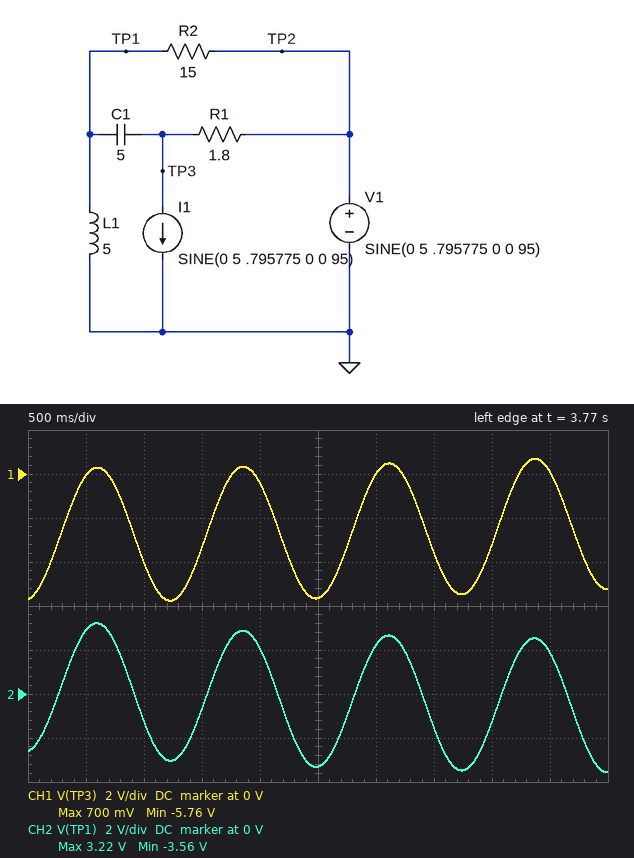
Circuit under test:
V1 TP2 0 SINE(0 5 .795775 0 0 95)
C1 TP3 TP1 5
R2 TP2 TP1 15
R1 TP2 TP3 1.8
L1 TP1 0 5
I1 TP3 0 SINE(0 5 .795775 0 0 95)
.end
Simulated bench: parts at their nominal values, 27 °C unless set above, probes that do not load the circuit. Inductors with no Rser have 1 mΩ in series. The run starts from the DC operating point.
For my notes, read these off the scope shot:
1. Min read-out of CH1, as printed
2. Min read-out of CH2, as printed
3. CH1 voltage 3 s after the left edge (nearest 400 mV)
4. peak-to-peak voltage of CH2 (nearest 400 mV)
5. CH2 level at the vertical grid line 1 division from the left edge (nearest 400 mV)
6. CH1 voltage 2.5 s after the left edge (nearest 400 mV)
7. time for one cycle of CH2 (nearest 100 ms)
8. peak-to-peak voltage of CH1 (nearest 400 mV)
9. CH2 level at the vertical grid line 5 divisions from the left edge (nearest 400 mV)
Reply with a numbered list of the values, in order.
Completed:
1. -5.76 V
2. -3.56 V
3. 0 V
4. 6.8 V
5. 2.8 V
6. -5.6 V
7. 1.3 s
8. 6.4 V
9. -3.2 V
